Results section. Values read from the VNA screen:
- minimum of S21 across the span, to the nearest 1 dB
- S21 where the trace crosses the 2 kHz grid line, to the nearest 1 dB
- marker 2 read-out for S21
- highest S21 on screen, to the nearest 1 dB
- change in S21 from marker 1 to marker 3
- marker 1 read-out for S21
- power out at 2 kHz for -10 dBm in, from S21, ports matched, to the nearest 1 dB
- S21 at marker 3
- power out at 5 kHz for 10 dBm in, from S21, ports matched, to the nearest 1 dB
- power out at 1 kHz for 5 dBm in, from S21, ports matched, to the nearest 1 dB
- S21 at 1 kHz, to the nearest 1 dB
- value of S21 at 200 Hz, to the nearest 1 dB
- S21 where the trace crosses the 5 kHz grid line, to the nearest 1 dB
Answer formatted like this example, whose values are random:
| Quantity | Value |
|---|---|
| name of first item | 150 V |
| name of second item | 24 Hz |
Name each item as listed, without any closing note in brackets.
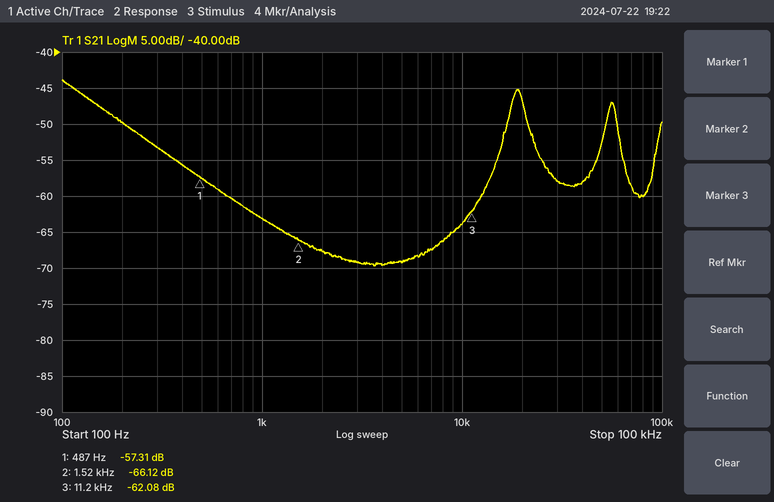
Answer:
| Quantity | Value |
|---|---|
| minimum of S21 across the span, to the nearest 1 dB | -70 dB |
| S21 where the trace crosses the 2 kHz grid line, to the nearest 1 dB | -68 dB |
| marker 2 read-out for S21 | -66.12 dB |
| highest S21 on screen, to the nearest 1 dB | -44 dB |
| change in S21 from marker 1 to marker 3 | -4.77 dB |
| marker 1 read-out for S21 | -57.31 dB |
| power out at 2 kHz for -10 dBm in, from S21, ports matched, to the nearest 1 dB | -78 dBm |
| S21 at marker 3 | -62.08 dB |
| power out at 5 kHz for 10 dBm in, from S21, ports matched, to the nearest 1 dB | -59 dBm |
| power out at 1 kHz for 5 dBm in, from S21, ports matched, to the nearest 1 dB | -58 dBm |
| S21 at 1 kHz, to the nearest 1 dB | -63 dB |
| value of S21 at 200 Hz, to the nearest 1 dB | -50 dB |
| S21 where the trace crosses the 5 kHz grid line, to the nearest 1 dB | -69 dB |
